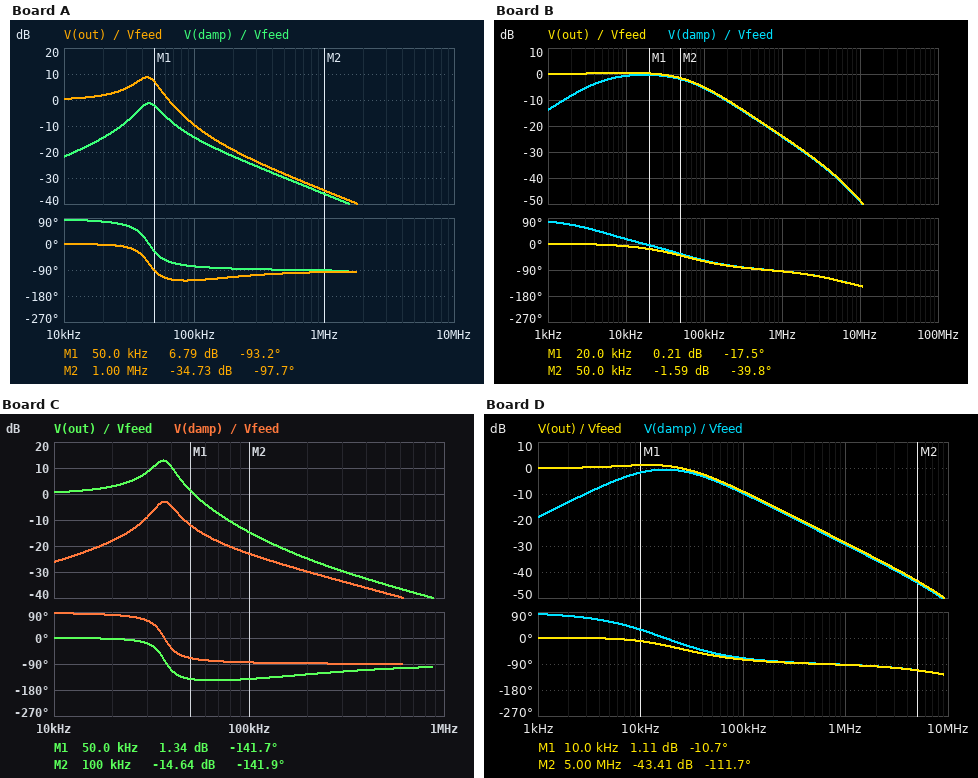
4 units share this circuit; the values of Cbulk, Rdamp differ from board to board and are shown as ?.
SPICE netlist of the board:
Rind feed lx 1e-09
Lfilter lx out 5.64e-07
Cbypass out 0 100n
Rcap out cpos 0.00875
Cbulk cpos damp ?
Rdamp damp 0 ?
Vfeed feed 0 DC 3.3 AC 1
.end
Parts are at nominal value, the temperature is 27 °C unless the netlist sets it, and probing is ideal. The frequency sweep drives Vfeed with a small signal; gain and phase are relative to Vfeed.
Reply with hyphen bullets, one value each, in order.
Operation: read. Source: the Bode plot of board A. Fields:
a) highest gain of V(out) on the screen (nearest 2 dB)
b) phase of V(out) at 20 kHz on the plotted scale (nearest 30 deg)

- 8 dB
- 0 deg
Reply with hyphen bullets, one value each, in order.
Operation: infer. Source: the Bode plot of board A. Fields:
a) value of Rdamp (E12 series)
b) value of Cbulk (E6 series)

- 0.056 Ω
- 22 µF
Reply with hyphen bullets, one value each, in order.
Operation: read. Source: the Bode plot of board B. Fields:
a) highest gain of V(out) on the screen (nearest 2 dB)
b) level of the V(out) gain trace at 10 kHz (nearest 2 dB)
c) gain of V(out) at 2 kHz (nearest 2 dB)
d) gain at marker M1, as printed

- 0 dB
- 0 dB
- 0 dB
- 0.21 dB
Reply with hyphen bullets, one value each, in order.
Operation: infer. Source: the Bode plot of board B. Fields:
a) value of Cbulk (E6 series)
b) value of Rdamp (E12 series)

- 150 µF
- 0.22 Ω
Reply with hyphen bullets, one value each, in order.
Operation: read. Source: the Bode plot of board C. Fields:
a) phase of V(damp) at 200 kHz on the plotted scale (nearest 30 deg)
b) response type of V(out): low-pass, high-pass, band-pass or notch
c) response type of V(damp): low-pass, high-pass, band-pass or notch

- -90 deg
- low-pass
- band-pass
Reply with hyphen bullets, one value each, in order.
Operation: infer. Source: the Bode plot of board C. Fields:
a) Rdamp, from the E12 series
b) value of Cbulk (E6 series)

- 0.022 Ω
- 33 µF
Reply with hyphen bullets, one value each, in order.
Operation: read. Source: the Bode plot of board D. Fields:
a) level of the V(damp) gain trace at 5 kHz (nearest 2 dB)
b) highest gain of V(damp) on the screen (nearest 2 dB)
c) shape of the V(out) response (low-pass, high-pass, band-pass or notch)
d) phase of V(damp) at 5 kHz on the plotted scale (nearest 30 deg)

- -6 dB
- 0 dB
- low-pass
- 60 deg
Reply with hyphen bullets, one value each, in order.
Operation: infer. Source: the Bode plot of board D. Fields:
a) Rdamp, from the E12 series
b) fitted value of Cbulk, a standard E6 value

- 0.12 Ω
- 150 µF
